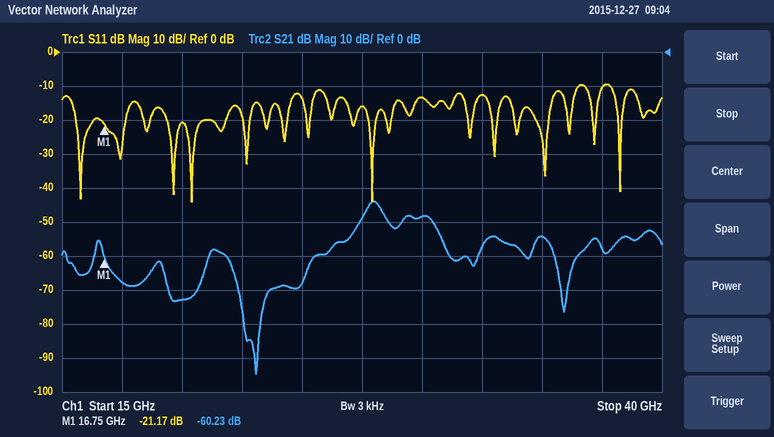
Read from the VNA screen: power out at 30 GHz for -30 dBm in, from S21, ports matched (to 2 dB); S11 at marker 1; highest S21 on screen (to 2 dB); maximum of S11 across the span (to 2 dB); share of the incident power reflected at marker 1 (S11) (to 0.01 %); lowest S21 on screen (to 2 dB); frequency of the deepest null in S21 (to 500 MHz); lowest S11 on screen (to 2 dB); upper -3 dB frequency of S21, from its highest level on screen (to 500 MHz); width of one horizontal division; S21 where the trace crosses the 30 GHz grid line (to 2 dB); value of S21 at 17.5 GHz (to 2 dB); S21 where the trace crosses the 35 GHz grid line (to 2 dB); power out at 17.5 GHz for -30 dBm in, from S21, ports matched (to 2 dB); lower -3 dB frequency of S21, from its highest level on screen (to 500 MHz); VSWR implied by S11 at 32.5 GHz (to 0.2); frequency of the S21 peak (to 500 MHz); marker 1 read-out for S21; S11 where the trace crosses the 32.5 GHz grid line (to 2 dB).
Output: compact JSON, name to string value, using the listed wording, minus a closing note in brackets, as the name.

{"power out at 30 GHz for -30 dBm in, from S21, ports matched": "-78 dBm", "S11 at marker 1": "-21.17 dB", "highest S21 on screen": "-44 dB", "maximum of S11 across the span": "-10 dB", "share of the incident power reflected at marker 1 (S11)": "0.76 %", "lowest S21 on screen": "-94 dB", "frequency of the deepest null in S21": "23.0 GHz", "lowest S11 on screen": "-44 dB", "upper -3 dB frequency of S21, from its highest level on screen": "28.5 GHz", "width of one horizontal division": "2.5 GHz", "S21 where the trace crosses the 30 GHz grid line": "-48 dB", "value of S21 at 17.5 GHz": "-68 dB", "S21 where the trace crosses the 35 GHz grid line": "-54 dB", "power out at 17.5 GHz for -30 dBm in, from S21, ports matched": "-98 dBm", "lower -3 dB frequency of S21, from its highest level on screen": "27.5 GHz", "VSWR implied by S11 at 32.5 GHz": "1.6", "frequency of the S21 peak": "28.0 GHz", "marker 1 read-out for S21": "-60.23 dB", "S11 where the trace crosses the 32.5 GHz grid line": "-12 dB"}
